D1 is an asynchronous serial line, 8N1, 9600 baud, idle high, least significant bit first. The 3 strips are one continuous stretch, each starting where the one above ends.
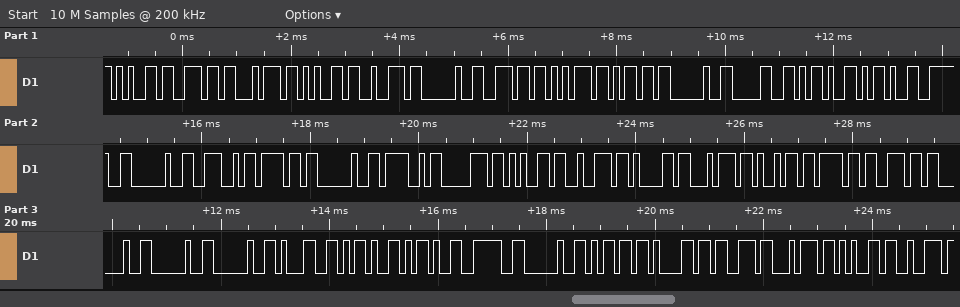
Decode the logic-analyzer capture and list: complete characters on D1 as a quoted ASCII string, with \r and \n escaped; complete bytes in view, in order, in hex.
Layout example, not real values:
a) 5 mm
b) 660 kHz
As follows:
a) "enter num 0--> No Operation   1--> master"
b) 65 6E 74 65 72 20 6E 75 6D 20 30 2D 2D 3E 20 4E 6F 20 4F 70 65 72 61 74 69 6F 6E 20 20 20 31 2D 2D 3E 20 6D 61 73 74 65 72
